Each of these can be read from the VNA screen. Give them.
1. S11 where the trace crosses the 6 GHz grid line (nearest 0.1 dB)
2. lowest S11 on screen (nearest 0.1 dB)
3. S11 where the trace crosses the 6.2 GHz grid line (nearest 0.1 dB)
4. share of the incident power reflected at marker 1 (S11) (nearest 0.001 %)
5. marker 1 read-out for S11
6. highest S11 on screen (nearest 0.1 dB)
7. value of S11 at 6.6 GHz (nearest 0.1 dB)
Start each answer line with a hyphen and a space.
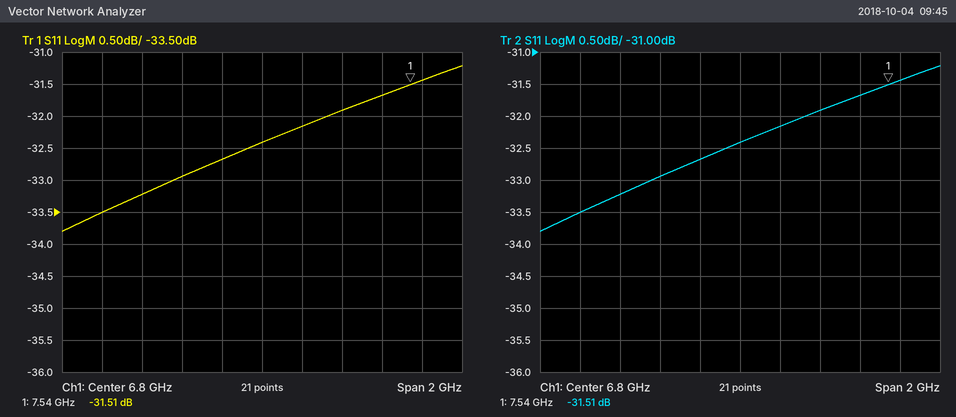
- -33.5 dB
- -33.8 dB
- -33.2 dB
- 0.071 %
- -31.51 dB
- -31.2 dB
- -32.7 dB
